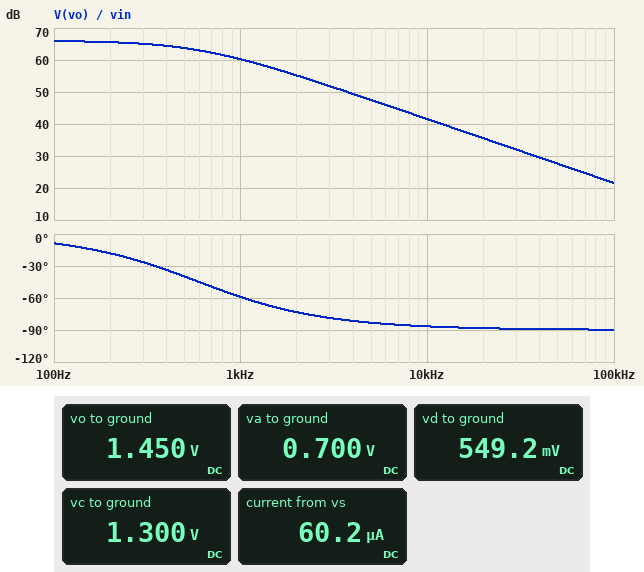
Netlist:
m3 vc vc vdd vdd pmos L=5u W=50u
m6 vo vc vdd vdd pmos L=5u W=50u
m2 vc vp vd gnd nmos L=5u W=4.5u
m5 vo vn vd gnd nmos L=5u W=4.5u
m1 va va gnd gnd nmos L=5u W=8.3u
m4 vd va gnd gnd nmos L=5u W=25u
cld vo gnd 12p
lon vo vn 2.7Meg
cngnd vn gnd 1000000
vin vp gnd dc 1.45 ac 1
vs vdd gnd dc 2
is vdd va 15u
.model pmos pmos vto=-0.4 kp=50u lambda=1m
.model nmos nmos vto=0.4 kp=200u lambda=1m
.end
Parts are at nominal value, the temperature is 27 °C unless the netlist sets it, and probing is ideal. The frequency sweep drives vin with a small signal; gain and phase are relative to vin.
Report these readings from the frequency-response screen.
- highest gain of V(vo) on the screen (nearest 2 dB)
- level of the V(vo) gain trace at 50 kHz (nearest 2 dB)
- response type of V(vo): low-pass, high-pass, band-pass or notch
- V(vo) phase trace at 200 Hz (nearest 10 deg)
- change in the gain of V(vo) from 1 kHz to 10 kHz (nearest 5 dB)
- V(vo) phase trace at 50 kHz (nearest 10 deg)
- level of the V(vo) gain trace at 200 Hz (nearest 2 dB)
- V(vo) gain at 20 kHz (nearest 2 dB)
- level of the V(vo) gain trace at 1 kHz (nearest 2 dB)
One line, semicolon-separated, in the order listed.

66 dB; 28 dB; low-pass; -20 deg; -20 dB; -90 deg; 66 dB; 36 dB; 60 dB
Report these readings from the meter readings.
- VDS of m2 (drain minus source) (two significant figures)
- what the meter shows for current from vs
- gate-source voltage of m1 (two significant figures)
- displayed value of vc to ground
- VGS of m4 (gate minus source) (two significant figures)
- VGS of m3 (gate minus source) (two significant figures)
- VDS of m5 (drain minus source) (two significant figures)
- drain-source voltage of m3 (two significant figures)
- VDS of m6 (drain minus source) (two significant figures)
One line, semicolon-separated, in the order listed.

750 mV; 60.2 µA; 700 mV; 1.300 V; 700 mV; -700 mV; 900 mV; -700 mV; -550 mV
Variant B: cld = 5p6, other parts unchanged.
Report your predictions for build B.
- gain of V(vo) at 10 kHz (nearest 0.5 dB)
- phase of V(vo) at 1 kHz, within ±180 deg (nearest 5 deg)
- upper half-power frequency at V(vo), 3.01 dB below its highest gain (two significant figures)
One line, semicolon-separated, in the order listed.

48.0 dB; -40 deg; 1.3 kHz
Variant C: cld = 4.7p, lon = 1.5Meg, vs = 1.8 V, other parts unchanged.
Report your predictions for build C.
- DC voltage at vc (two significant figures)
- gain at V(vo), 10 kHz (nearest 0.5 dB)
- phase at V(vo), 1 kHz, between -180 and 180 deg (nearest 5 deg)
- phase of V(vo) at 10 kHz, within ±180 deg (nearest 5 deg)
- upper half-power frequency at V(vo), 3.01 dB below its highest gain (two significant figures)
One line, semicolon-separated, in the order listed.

1.1 V; 49.5 dB; -35 deg; -80 deg; 1.5 kHz
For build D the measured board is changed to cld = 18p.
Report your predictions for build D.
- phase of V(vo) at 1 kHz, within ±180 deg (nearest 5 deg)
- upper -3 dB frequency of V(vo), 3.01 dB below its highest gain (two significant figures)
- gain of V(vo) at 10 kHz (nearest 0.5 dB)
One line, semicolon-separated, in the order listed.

-70 deg; 400 Hz; 38.0 dB
